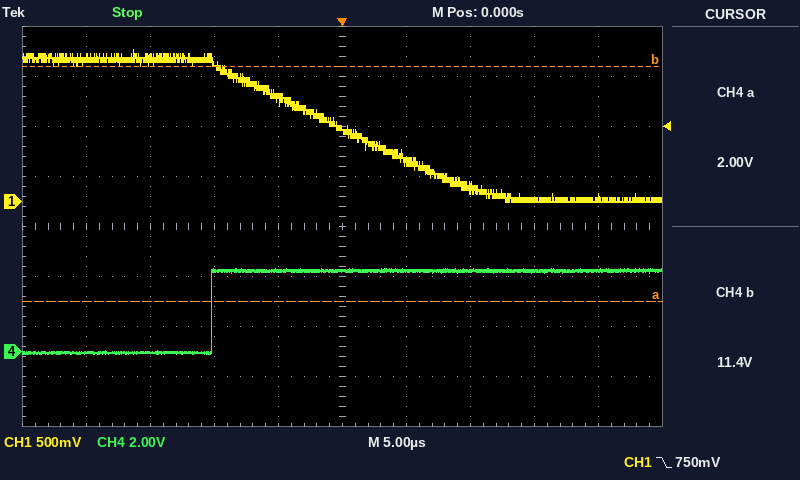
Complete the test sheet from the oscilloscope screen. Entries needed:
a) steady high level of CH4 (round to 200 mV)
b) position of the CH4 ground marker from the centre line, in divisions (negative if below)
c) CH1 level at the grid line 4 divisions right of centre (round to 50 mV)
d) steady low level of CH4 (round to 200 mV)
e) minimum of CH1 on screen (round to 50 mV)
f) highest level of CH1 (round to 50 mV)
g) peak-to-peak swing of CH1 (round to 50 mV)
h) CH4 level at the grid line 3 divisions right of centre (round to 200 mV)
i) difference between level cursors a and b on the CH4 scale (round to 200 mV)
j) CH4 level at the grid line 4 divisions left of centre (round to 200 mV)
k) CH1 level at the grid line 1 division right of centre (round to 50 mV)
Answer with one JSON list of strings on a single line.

["3.2 V", "-2.5 div", "50 mV", "0.0 V", "0 mV", "1.50 V", "1.50 V", "3.2 V", "9.4 V", "0.0 V", "400 mV"]
